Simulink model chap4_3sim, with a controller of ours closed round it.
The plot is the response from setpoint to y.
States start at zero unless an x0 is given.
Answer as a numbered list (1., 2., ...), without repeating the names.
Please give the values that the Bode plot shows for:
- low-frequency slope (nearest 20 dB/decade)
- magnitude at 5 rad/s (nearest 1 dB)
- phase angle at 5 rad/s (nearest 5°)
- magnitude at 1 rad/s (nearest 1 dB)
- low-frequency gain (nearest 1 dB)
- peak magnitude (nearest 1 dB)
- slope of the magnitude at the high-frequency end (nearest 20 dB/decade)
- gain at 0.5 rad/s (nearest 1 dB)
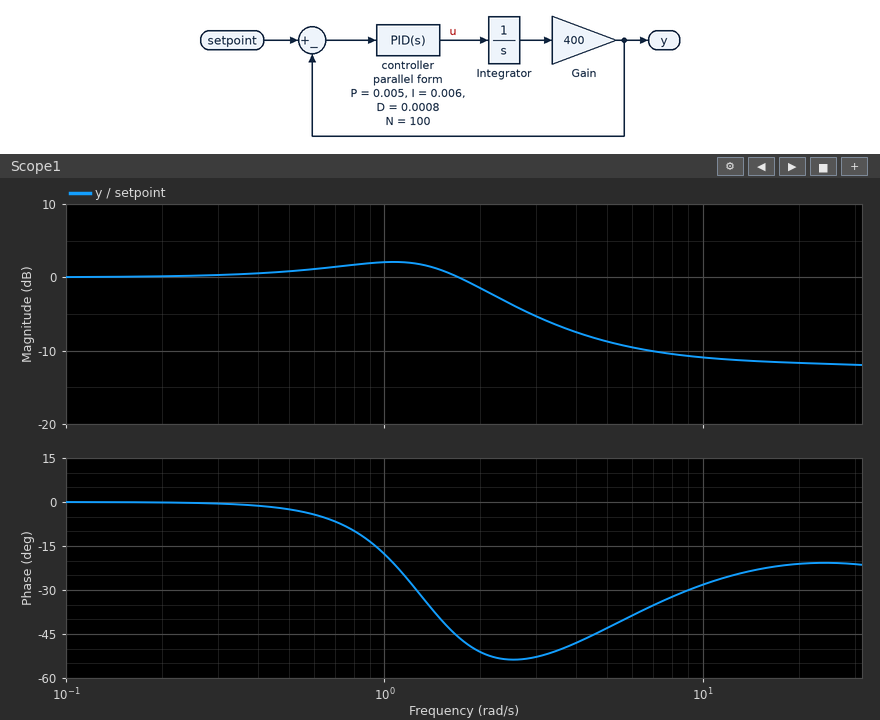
1. 0 dB/decade
2. -9 dB
3. -45°
4. 2 dB
5. 0 dB
6. 2 dB
7. 0 dB/decade
8. 1 dB
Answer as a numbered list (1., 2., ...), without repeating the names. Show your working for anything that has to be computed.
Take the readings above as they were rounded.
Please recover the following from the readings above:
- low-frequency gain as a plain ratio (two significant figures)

1. 10^(0 / 20) = 1.0
